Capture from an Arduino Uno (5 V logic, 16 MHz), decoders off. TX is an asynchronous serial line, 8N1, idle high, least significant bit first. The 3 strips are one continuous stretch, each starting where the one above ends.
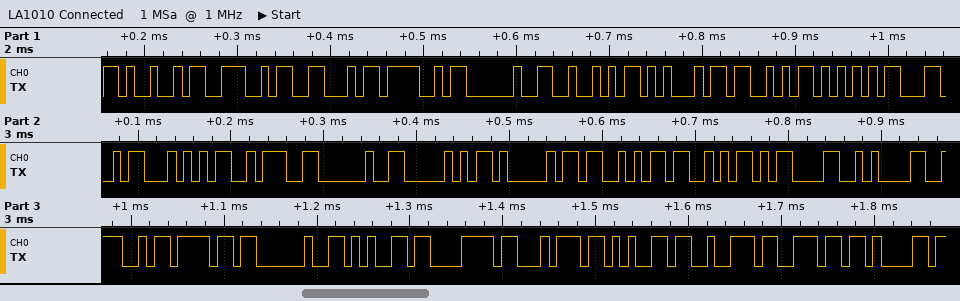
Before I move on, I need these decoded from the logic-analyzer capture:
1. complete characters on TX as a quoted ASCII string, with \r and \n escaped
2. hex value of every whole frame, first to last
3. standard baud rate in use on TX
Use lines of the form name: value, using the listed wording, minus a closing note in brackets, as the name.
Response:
complete characters on TX as a quoted ASCII string, with \r and \n escaped: "INFO RESULT: PASS\r\nNo externa"
hex value of every whole frame, first to last: 49 4E 46 4F 20 52 45 53 55 4C 54 3A 20 50 41 53 53 0D 0A 4E 6F 20 65 78 74 65 72 6E 61
standard baud rate in use on TX: 115200 baud
